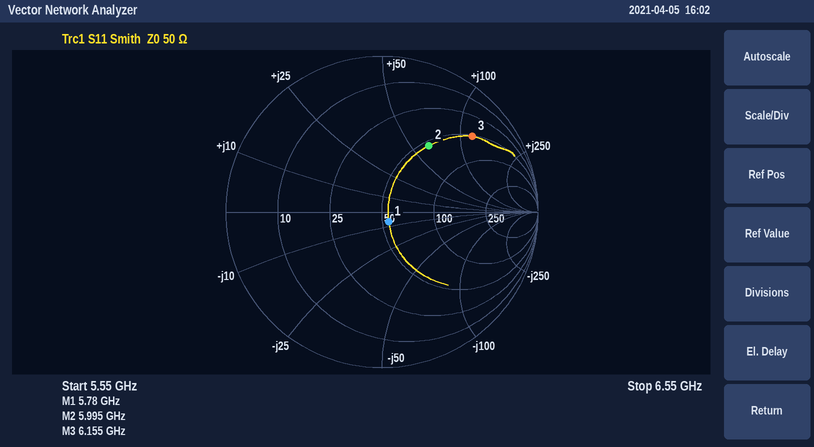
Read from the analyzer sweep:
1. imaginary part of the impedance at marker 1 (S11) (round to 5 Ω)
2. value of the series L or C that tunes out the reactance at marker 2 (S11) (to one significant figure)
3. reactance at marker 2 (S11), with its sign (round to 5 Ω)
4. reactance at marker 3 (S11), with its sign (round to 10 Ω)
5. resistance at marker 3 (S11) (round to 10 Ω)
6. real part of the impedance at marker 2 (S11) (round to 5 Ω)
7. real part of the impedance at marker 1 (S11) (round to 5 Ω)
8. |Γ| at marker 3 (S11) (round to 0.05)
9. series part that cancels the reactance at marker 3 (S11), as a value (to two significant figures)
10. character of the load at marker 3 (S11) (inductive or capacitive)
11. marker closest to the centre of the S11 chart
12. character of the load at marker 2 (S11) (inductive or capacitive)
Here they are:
-5 Ω
400 fF
+65 Ω
+120 Ω
50 Ω
55 Ω
55 Ω
0.75
220 fF
inductive
marker 1
inductive
